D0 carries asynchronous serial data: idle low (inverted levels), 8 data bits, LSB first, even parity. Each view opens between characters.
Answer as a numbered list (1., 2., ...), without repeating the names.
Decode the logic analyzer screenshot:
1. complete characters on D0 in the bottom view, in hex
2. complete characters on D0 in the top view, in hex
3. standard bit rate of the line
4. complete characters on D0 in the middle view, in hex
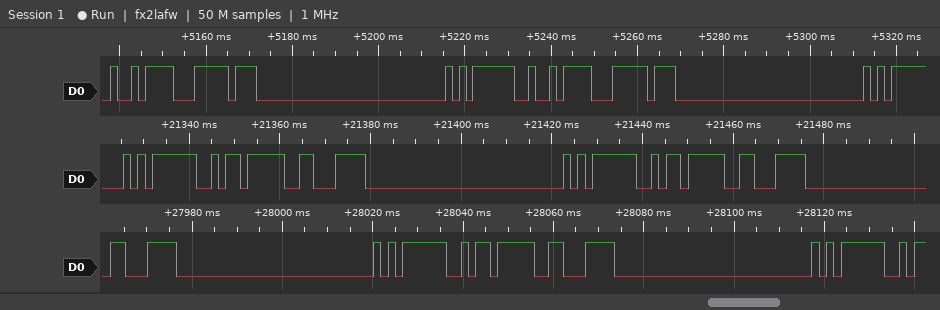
1. 0E, 05, 09, 0E, 05
2. 0B, 10, 05, 0B, 10
3. 600 baud
4. 05, 09, 0E, 05, 09, 0E
